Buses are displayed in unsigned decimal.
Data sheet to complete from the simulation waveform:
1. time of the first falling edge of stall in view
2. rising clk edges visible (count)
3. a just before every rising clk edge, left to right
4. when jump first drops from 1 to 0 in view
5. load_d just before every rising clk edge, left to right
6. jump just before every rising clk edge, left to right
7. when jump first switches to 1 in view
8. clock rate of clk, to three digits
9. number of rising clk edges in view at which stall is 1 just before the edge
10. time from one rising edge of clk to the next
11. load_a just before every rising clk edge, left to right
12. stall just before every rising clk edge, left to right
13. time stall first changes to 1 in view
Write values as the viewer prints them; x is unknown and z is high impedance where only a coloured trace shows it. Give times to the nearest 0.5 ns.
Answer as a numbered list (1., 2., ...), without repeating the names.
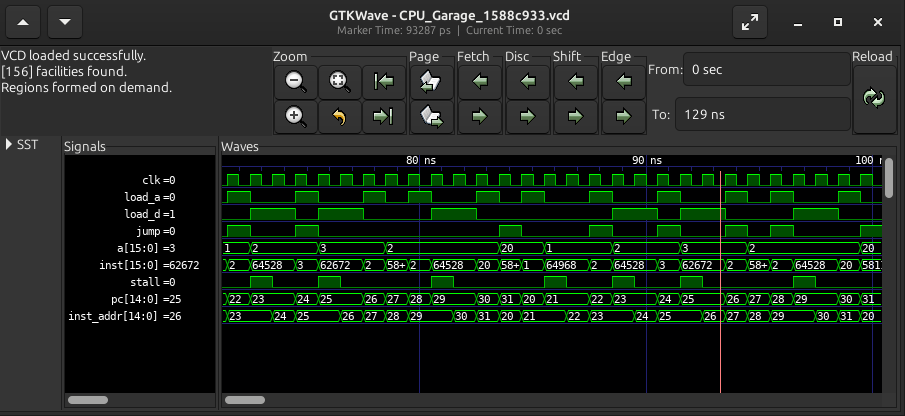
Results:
1. 73.5 ns
2. 29
3. 1, 1, 2, 2, 2, 3, 3, 3, 2, 2, 2, 2, 2, 20, 20, 1, 1, 1, 2, 2, 2, 3, 3, 3, 2, 2, 2, 2, 2
4. 72.5 ns
5. 0 0 1 1 0 1 1 0 0 0 1 1 0 0 0 0 0 0 1 1 0 1 1 0 0 0 1 1 0
6. 0 1 0 0 1 0 0 0 0 0 0 0 0 1 0 0 0 1 0 0 1 0 0 1 0 1 0 0 0
7. 71.5 ns
8. 1.00 GHz
9. 7
10. 1 ns
11. 0 1 0 0 1 0 0 1 0 1 0 0 1 0 1 0 0 1 0 0 1 0 0 1 0 1 0 0 1
12. 0 0 1 0 0 1 0 0 0 0 1 0 0 0 0 1 0 0 1 0 0 1 0 0 0 0 1 0 0
13. 72.5 ns
